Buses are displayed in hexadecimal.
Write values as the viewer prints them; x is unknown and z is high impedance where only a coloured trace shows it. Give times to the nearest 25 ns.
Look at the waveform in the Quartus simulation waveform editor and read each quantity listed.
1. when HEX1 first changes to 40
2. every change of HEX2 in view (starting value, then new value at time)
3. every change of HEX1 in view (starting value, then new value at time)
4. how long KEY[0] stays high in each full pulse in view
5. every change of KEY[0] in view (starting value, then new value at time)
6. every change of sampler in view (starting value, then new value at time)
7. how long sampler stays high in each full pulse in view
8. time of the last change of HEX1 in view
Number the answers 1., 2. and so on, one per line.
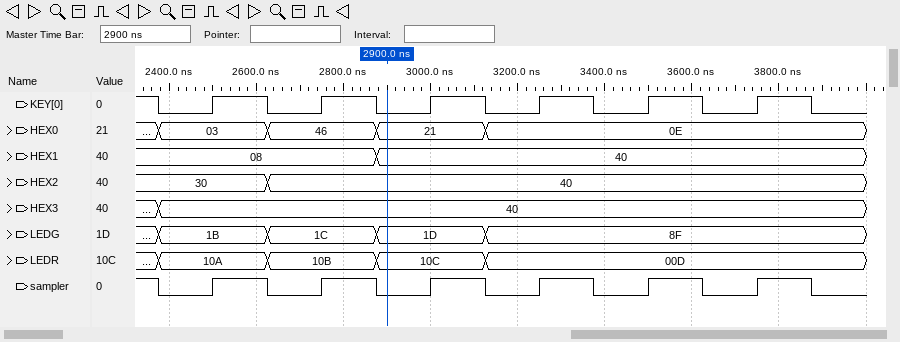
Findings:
1. 2875 ns
2. 30, 40 at 2625 ns
3. 08, 40 at 2875 ns
4. 125 ns, 125 ns, 125 ns, 125 ns, 125 ns, 125 ns
5. 1, 0 at 2375 ns, 1 at 2500 ns, 0 at 2625 ns, 1 at 2750 ns, 0 at 2875 ns, 1 at 3000 ns, 0 at 3125 ns, 1 at 3250 ns, 0 at 3375 ns, 1 at 3500 ns, 0 at 3625 ns, 1 at 3750 ns, 0 at 3875 ns
6. 1, 0 at 2375 ns, 1 at 2500 ns, 0 at 2625 ns, 1 at 2750 ns, 0 at 2875 ns, 1 at 3000 ns, 0 at 3125 ns, 1 at 3250 ns, 0 at 3375 ns, 1 at 3500 ns, 0 at 3625 ns, 1 at 3750 ns, 0 at 3875 ns
7. 125 ns, 125 ns, 125 ns, 125 ns, 125 ns, 125 ns
8. 2875 ns
